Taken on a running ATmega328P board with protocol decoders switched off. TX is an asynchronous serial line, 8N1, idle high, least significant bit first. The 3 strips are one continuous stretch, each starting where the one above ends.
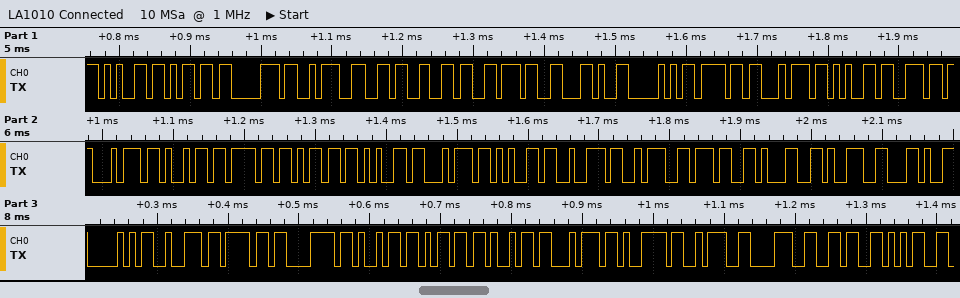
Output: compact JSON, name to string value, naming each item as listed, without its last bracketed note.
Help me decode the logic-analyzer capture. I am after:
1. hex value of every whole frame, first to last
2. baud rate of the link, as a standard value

{"hex value of every whole frame, first to last": "65 6D 70 3A 36 36 37 2C 50 6F 74 65 6E 74 69 6F 6D 65 74 65 72 3A 37 31 39 2C 50 72 6F 78 69 6D 69 74 79 3A 38 36 35", "baud rate of the link, as a standard value": "115200 baud"}
